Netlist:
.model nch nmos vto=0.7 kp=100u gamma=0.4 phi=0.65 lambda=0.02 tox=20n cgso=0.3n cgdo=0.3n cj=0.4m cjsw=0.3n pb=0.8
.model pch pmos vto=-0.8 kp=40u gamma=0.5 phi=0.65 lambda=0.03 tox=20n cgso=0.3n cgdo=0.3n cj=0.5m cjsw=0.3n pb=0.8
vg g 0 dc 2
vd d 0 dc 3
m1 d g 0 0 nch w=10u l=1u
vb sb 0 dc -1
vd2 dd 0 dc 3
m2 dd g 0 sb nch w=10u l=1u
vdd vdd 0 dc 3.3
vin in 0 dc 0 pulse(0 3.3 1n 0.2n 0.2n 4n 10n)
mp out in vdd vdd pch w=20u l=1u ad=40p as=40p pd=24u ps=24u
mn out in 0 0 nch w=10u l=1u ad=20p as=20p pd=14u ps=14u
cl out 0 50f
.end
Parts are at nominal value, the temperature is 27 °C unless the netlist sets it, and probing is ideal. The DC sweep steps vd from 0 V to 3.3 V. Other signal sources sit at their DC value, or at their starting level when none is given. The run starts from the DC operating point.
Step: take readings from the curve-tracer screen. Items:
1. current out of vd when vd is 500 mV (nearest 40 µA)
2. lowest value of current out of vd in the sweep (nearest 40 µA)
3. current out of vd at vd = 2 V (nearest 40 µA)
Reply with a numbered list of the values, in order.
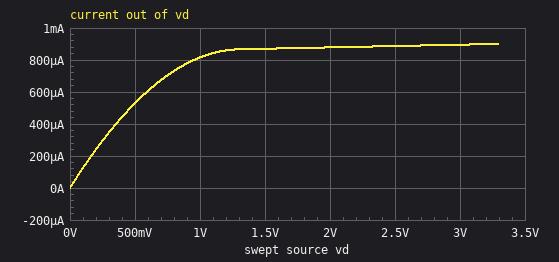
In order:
1. 520 µA
2. 0 A
3. 880 µA
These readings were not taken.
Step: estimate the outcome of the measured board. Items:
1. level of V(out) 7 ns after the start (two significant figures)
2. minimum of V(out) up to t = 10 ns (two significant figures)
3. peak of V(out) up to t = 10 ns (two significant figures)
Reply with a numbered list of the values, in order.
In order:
1. 3.3 V
2. -120 mV
3. 3.5 V
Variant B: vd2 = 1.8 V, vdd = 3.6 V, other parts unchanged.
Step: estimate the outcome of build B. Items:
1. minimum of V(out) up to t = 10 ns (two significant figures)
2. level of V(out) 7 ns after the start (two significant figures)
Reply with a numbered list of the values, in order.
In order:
1. -98 mV
2. 3.6 V
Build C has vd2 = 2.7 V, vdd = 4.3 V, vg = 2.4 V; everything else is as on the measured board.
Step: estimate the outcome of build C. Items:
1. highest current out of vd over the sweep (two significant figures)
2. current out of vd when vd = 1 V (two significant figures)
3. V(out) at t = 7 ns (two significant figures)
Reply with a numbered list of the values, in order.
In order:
1. 1.5 mA
2. 1.2 mA
3. 4.3 V
